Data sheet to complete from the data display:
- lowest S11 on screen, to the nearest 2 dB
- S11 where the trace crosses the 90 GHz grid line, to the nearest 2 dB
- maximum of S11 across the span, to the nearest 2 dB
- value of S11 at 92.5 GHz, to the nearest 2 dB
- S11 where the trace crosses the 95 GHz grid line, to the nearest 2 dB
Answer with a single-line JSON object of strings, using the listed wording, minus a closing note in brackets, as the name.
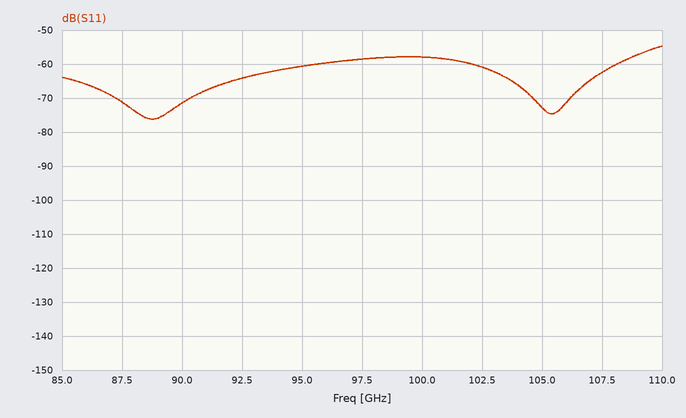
{"lowest S11 on screen, to the nearest 2 dB": "-76 dB", "S11 where the trace crosses the 90 GHz grid line, to the nearest 2 dB": "-72 dB", "maximum of S11 across the span, to the nearest 2 dB": "-54 dB", "value of S11 at 92.5 GHz, to the nearest 2 dB": "-64 dB", "S11 where the trace crosses the 95 GHz grid line, to the nearest 2 dB": "-60 dB"}
